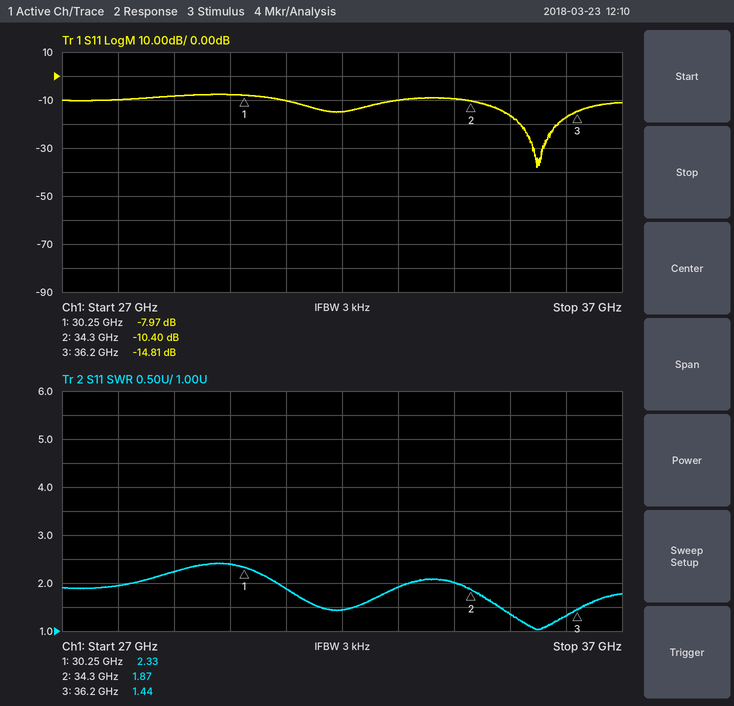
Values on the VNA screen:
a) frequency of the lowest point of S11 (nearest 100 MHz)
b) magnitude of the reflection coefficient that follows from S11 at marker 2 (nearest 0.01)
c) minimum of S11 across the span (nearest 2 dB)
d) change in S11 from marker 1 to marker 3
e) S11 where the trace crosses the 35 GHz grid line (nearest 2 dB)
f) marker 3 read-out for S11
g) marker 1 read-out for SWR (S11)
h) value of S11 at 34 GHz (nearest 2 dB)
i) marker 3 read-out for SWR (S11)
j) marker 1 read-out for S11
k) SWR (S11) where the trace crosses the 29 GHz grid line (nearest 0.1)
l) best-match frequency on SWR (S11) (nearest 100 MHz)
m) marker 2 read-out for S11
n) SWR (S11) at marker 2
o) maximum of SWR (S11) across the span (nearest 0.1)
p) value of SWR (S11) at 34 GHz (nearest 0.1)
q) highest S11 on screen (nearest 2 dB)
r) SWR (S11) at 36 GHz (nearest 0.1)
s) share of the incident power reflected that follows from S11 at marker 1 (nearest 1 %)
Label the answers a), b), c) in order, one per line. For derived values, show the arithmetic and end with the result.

a) 35.5 GHz
b) 10^(-10.4/20) ≈ 0.30
c) -38 dB
d) -14.81 − (-7.97) = -6.84 dB
e) -16 dB
f) -14.81 dB
g) 2.33
h) -10 dB
i) 1.44
j) -7.97 dB
k) 2.2
l) 35.5 GHz
m) -10.40 dB
n) 1.87
o) 2.4
p) 2.0
q) -8 dB
r) 1.3
s) 10^(-7.97/10) ≈ 16 %
